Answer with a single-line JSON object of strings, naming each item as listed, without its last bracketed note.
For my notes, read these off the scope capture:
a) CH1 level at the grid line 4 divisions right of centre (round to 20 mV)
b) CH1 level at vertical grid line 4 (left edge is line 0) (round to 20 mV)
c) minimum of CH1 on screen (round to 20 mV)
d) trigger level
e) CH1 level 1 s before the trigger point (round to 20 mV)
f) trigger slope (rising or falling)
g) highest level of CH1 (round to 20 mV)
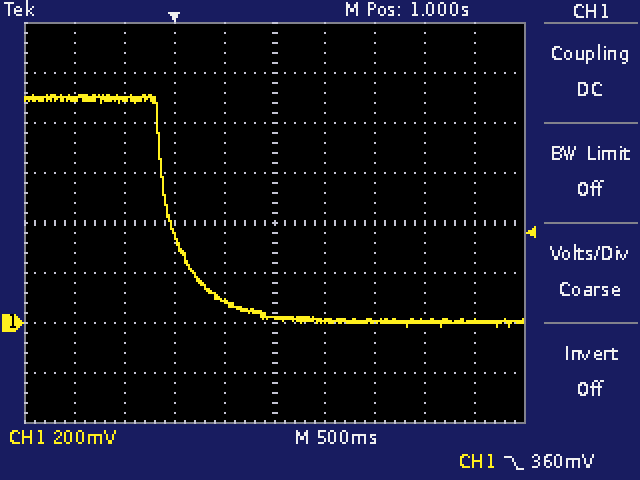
{"CH1 level at the grid line 4 divisions right of centre": "0 mV", "CH1 level at vertical grid line 4 (left edge is line 0)": "80 mV", "minimum of CH1 on screen": "-20 mV", "trigger level": "360 mV", "CH1 level 1 s before the trigger point": "900 mV", "trigger slope": "falling", "highest level of CH1": "920 mV"}
